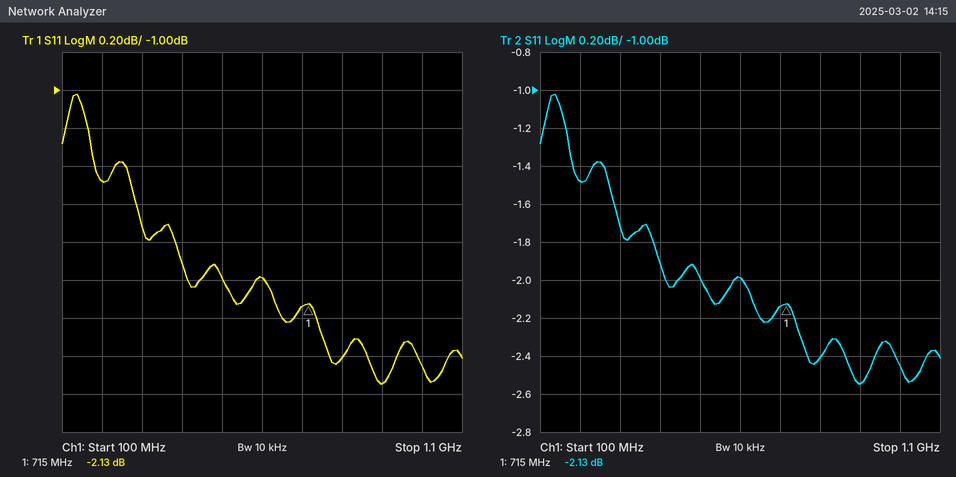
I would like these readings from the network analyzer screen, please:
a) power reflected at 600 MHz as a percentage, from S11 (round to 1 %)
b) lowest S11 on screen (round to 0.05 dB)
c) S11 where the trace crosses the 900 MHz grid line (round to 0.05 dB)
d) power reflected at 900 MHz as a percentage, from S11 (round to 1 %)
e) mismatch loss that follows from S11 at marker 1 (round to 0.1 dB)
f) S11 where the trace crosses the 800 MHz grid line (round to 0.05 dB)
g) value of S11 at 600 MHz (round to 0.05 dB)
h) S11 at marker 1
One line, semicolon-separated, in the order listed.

63 %; -2.55 dB; -2.55 dB; 56 %; 4.1 dB; -2.40 dB; -2.00 dB; -2.13 dB
